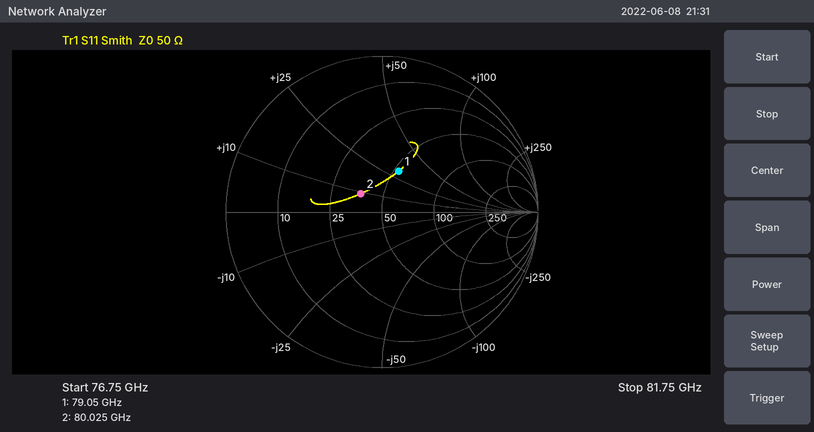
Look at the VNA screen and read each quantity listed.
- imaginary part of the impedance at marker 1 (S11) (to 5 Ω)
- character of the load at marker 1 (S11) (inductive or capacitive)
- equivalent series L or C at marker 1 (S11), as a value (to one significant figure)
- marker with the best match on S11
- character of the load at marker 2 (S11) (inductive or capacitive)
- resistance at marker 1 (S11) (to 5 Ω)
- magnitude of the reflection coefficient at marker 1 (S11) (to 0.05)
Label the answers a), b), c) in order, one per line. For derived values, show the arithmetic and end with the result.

a) +30 Ω
b) inductive
c) L = 30 Ω/(2π × 79.05 GHz) ≈ 60 pH
d) marker 2
e) inductive
f) 55 Ω
g) 0.30
